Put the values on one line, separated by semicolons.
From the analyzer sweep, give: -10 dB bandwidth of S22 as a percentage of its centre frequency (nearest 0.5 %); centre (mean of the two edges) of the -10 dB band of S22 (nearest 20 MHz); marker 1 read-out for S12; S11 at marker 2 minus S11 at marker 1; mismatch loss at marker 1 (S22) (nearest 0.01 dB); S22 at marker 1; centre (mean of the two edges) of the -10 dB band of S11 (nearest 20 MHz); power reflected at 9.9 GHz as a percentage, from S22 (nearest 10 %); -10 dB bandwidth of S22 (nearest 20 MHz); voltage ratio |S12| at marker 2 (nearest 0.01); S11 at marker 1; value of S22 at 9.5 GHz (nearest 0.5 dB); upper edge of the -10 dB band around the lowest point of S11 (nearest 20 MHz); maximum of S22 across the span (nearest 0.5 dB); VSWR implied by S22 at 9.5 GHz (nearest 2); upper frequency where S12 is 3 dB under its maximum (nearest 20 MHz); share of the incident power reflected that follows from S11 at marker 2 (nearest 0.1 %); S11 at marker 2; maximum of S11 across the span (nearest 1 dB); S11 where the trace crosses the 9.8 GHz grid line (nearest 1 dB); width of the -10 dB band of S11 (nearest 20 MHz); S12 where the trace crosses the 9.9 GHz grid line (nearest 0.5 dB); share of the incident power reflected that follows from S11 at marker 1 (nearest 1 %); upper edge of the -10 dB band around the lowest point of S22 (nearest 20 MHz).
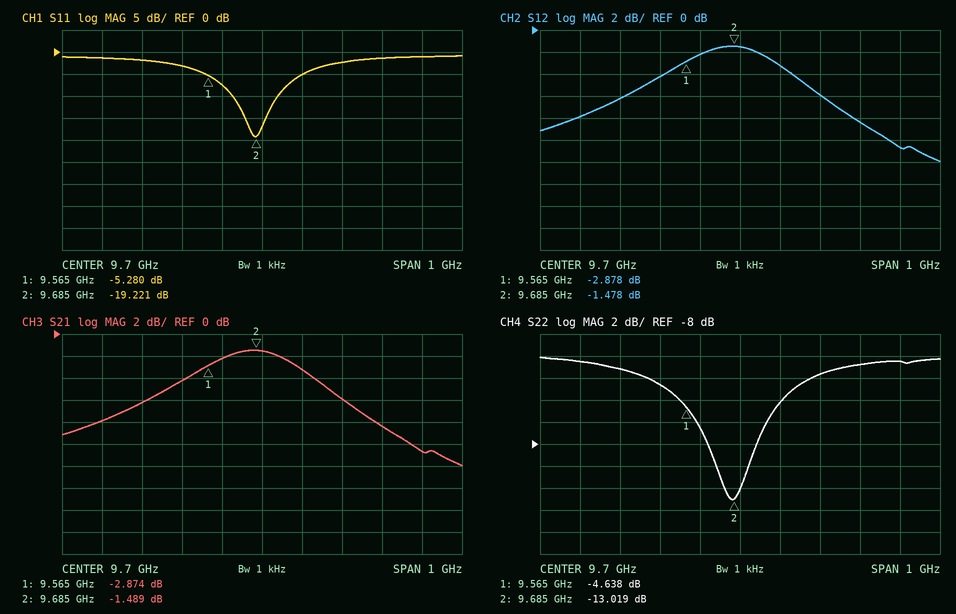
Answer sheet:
1.0 %; 9.68 GHz; -2.878 dB; -13.941 dB; 1.83 dB; -4.638 dB; 9.68 GHz; 70 %; 80 MHz; 0.84; -5.280 dB; -2.5 dB; 9.74 GHz; 0.0 dB; 6; 9.84 GHz; 1.2 %; -19.221 dB; -1 dB; -5 dB; 120 MHz; -6.0 dB; 30 %; 9.72 GHz
